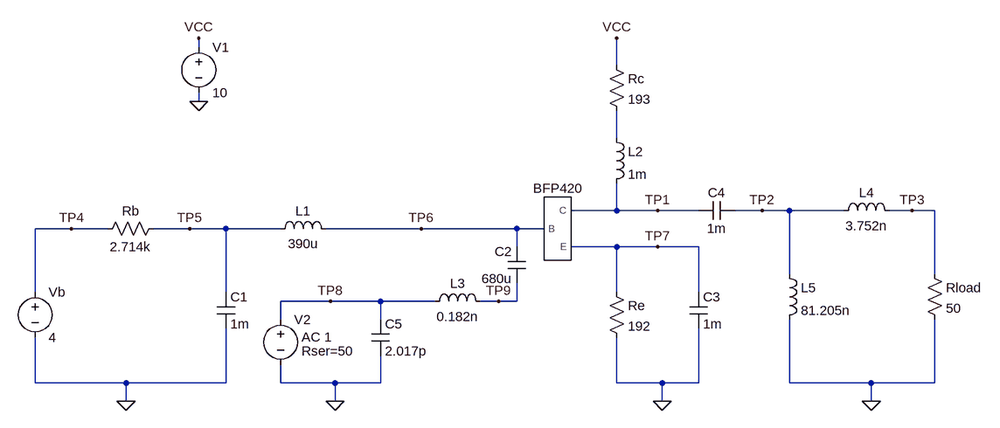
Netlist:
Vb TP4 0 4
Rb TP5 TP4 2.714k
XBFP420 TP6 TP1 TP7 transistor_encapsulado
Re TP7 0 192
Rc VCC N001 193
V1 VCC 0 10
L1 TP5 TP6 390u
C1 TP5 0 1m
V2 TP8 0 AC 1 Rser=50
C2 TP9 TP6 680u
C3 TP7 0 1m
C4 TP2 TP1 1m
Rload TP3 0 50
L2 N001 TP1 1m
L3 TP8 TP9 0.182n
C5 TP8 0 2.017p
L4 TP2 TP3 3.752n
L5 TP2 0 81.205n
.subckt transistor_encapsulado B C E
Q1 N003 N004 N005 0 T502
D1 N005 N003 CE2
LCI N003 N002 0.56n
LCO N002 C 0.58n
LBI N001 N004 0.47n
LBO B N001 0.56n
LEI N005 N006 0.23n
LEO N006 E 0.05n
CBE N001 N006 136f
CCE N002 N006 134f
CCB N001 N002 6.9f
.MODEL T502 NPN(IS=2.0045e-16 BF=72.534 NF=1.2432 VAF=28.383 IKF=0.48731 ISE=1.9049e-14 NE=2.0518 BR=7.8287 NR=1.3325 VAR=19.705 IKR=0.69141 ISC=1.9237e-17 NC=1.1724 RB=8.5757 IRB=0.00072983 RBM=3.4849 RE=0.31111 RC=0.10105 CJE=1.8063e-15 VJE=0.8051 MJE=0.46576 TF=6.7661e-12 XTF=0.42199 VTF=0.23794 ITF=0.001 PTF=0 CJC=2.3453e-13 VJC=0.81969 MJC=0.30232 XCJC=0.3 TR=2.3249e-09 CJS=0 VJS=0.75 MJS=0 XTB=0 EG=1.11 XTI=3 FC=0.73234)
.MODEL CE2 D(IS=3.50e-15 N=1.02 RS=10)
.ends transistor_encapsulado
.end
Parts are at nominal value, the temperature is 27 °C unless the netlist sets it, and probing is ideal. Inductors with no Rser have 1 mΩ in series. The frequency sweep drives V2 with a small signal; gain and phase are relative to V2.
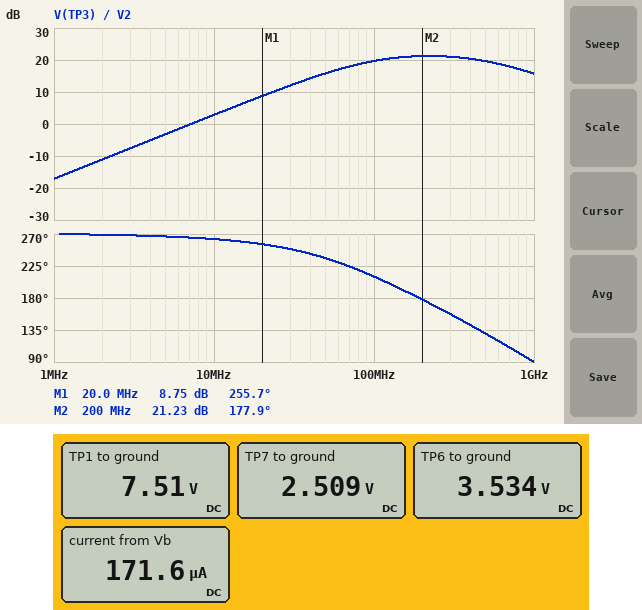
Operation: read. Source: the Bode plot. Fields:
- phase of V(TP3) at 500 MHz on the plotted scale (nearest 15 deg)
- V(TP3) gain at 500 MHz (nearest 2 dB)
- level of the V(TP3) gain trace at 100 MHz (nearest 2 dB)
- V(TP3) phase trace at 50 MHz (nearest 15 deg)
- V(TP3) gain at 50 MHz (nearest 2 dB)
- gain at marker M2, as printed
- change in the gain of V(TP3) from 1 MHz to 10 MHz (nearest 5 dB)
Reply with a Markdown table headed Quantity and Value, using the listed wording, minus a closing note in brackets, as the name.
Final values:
| Quantity | Value |
|---|---|
| phase of V(TP3) at 500 MHz on the plotted scale | 135 deg |
| V(TP3) gain at 500 MHz | 20 dB |
| level of the V(TP3) gain trace at 100 MHz | 20 dB |
| V(TP3) phase trace at 50 MHz | 240 deg |
| V(TP3) gain at 50 MHz | 16 dB |
| gain at marker M2, as printed | 21.23 dB |
| change in the gain of V(TP3) from 1 MHz to 10 MHz | 20 dB |
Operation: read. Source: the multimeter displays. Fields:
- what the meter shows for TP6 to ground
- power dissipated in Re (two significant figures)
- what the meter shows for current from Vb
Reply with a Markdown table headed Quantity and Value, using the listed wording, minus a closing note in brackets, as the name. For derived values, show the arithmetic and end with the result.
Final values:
| Quantity | Value |
|---|---|
| what the meter shows for TP6 to ground | 3.534 V |
| power dissipated in Re | (2.509 V)^2 / 192 Ω = 33 mW |
| what the meter shows for current from Vb | 171.6 µA |
